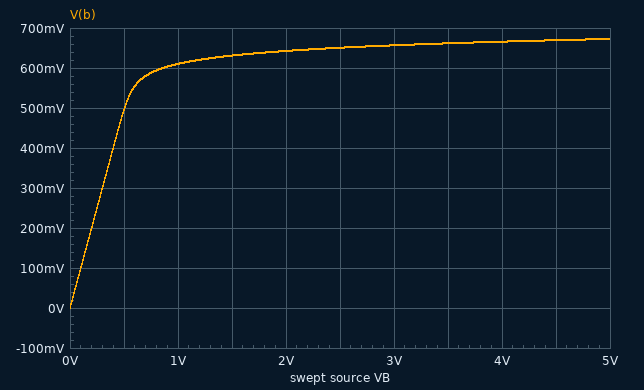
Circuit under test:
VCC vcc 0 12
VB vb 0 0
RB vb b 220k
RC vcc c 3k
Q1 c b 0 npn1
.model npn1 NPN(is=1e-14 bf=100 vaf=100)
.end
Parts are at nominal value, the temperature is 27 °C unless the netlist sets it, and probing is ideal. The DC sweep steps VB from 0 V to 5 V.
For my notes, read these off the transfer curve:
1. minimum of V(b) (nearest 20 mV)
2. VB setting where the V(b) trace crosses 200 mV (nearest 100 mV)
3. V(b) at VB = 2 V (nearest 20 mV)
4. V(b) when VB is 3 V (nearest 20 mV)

0 V
200 mV
640 mV
660 mV
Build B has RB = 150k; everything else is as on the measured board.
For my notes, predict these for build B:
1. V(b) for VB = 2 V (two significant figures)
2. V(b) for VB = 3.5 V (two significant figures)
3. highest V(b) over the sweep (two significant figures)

650 mV
670 mV
680 mV
